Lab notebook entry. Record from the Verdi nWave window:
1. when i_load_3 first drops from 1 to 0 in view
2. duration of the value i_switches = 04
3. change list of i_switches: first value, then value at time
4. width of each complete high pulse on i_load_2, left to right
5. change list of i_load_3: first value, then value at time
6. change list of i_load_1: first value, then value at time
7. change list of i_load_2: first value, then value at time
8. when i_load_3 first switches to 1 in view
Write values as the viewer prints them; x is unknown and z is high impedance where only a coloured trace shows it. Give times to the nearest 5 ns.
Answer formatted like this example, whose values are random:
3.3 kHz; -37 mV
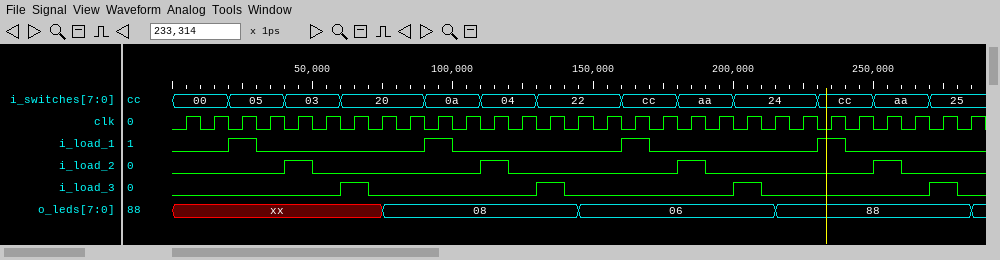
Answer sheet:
70 ns; 20 ns; 00, 05 at 20 ns, 03 at 40 ns, 20 at 60 ns, 0a at 90 ns, 04 at 110 ns, 22 at 130 ns, cc at 160 ns, aa at 180 ns, 24 at 200 ns, cc at 230 ns, aa at 250 ns, 25 at 270 ns; 10 ns, 10 ns, 10 ns, 10 ns; 0, 1 at 60 ns, 0 at 70 ns, 1 at 130 ns, 0 at 140 ns, 1 at 200 ns, 0 at 210 ns, 1 at 270 ns, 0 at 280 ns; 0, 1 at 20 ns, 0 at 30 ns, 1 at 90 ns, 0 at 100 ns, 1 at 160 ns, 0 at 170 ns, 1 at 230 ns, 0 at 240 ns; 0, 1 at 40 ns, 0 at 50 ns, 1 at 110 ns, 0 at 120 ns, 1 at 180 ns, 0 at 190 ns, 1 at 250 ns, 0 at 260 ns; 60 ns
